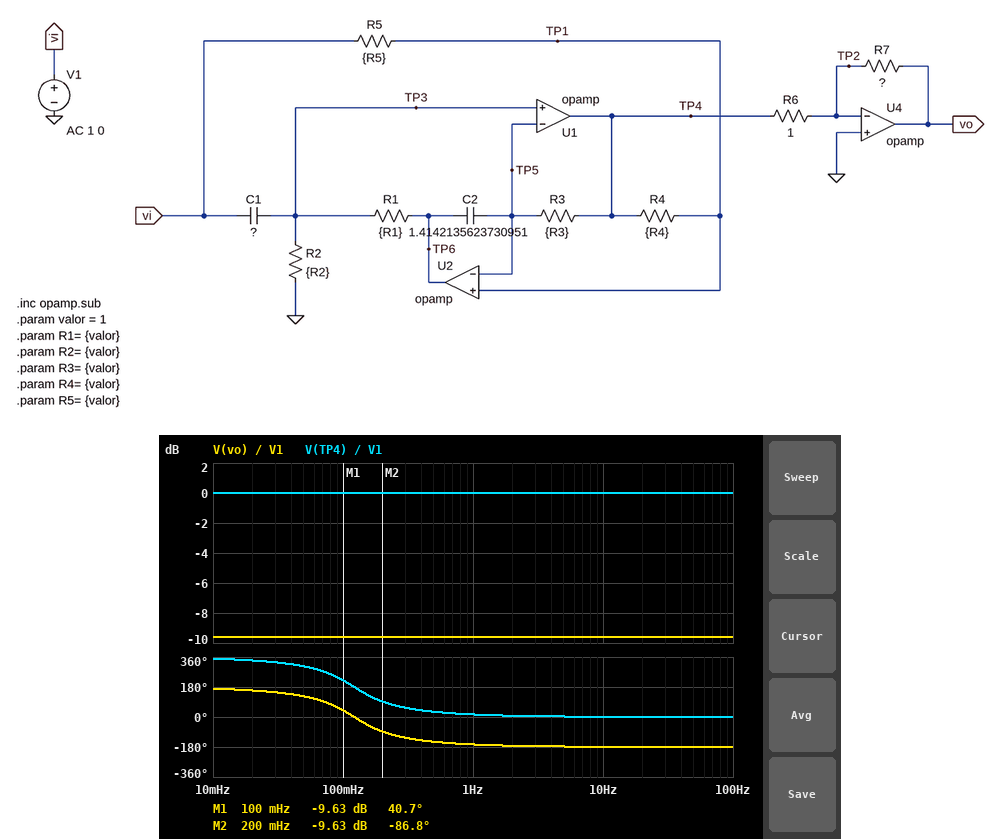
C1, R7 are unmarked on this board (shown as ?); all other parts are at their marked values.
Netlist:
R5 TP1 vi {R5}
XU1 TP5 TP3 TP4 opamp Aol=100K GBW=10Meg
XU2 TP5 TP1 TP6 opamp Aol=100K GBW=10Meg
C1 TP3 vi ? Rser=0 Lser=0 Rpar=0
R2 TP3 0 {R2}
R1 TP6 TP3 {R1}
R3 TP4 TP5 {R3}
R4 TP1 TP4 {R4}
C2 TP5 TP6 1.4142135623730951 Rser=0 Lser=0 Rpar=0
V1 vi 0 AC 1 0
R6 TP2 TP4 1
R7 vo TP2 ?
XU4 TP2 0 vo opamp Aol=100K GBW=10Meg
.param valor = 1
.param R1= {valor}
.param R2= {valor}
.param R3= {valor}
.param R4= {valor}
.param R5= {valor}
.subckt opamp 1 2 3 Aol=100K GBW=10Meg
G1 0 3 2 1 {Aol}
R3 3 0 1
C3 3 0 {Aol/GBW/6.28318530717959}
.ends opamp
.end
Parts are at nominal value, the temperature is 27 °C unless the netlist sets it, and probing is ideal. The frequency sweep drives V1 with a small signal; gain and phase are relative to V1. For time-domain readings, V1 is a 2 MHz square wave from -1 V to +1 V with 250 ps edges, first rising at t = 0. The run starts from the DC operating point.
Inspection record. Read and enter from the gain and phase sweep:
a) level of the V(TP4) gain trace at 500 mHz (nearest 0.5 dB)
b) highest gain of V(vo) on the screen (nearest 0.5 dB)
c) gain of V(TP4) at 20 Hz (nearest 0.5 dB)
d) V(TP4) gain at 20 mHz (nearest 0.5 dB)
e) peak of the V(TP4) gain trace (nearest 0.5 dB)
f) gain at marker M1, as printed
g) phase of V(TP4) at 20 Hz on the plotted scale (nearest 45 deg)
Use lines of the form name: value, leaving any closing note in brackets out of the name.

level of the V(TP4) gain trace at 500 mHz: 0 dB
highest gain of V(vo) on the screen: -9.5 dB
gain of V(TP4) at 20 Hz: 0 dB
V(TP4) gain at 20 mHz: 0 dB
peak of the V(TP4) gain trace: 0 dB
gain at marker M1, as printed: -9.63 dB
phase of V(TP4) at 20 Hz on the plotted scale: 0 deg
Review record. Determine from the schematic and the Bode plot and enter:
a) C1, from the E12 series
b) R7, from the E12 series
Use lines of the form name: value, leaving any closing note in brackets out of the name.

C1, from the E12 series: 1.2 F
R7, from the E12 series: 0.33 Ω
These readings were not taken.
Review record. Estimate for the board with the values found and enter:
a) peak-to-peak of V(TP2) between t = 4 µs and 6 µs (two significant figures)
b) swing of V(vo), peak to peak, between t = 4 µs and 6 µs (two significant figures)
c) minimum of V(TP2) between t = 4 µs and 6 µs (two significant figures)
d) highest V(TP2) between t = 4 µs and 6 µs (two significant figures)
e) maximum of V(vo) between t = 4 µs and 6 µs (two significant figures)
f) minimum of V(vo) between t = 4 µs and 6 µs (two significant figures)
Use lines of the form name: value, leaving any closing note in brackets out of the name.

peak-to-peak of V(TP2) between t = 4 µs and 6 µs: 530 mV
swing of V(vo), peak to peak, between t = 4 µs and 6 µs: 800 mV
minimum of V(TP2) between t = 4 µs and 6 µs: -270 mV
highest V(TP2) between t = 4 µs and 6 µs: 270 mV
maximum of V(vo) between t = 4 µs and 6 µs: 400 mV
minimum of V(vo) between t = 4 µs and 6 µs: -400 mV
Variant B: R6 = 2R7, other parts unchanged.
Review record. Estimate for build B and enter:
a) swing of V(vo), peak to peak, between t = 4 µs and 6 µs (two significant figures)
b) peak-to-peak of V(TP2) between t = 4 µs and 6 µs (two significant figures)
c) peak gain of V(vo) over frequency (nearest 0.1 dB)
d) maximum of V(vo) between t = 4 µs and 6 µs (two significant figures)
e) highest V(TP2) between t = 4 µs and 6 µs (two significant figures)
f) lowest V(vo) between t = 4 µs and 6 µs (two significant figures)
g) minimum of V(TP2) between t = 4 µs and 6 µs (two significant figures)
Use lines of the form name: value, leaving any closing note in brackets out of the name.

swing of V(vo), peak to peak, between t = 4 µs and 6 µs: 310 mV
peak-to-peak of V(TP2) between t = 4 µs and 6 µs: 210 mV
peak gain of V(vo) over frequency: -18.3 dB
maximum of V(vo) between t = 4 µs and 6 µs: 150 mV
highest V(TP2) between t = 4 µs and 6 µs: 110 mV
lowest V(vo) between t = 4 µs and 6 µs: -150 mV
minimum of V(TP2) between t = 4 µs and 6 µs: -110 mV
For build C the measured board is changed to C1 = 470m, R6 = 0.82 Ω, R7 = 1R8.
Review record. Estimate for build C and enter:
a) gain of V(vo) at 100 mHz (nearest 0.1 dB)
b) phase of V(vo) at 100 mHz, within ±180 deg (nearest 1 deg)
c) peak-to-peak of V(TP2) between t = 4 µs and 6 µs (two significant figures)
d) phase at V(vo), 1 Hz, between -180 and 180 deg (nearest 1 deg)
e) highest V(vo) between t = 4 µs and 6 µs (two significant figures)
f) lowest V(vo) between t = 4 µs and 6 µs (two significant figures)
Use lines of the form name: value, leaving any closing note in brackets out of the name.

gain of V(vo) at 100 mHz: 6.8 dB
phase of V(vo) at 100 mHz, within ±180 deg: 79 deg
peak-to-peak of V(TP2) between t = 4 µs and 6 µs: 2.1 V
phase at V(vo), 1 Hz, between -180 and 180 deg: -141 deg
highest V(vo) between t = 4 µs and 6 µs: 2.2 V
lowest V(vo) between t = 4 µs and 6 µs: -2.2 V
